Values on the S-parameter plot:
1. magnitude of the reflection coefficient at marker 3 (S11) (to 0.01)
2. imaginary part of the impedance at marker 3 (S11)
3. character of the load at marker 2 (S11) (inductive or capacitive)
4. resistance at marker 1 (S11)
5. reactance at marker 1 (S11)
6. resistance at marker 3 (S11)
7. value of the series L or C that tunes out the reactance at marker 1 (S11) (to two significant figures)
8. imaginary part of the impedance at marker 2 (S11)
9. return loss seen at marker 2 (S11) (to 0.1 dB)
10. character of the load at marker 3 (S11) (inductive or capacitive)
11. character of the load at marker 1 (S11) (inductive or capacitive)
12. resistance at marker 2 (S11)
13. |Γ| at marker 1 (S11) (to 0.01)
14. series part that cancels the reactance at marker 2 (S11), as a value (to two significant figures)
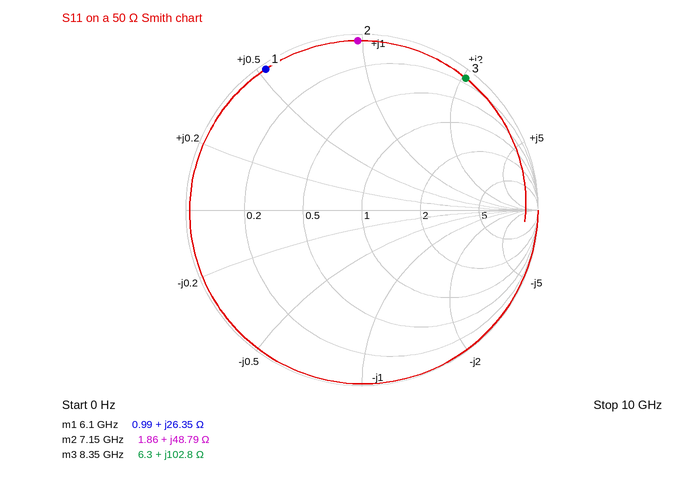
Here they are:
0.95
+102.8 Ω
inductive
0.99 Ω
+26.35 Ω
6.3 Ω
990 fF
+48.79 Ω
0.3 dB
inductive
inductive
1.86 Ω
0.97
460 fF
